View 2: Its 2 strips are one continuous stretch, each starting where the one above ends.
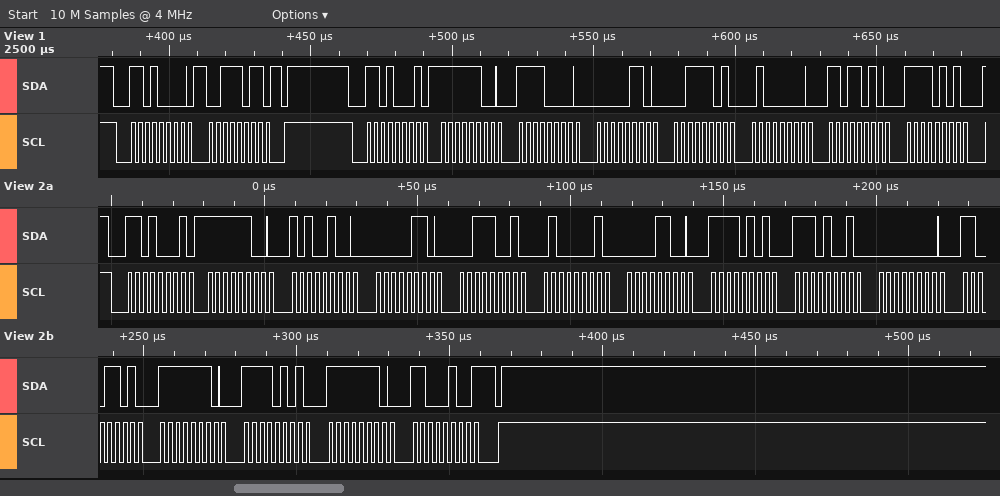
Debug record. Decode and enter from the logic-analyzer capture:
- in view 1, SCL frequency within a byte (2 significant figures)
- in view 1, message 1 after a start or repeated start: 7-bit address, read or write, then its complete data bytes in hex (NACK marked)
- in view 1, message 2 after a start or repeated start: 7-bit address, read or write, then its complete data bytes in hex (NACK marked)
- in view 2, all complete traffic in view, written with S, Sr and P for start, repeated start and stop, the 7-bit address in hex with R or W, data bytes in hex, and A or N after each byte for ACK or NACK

400 kHz
0x68 write: 3B
0x68 read: FC F0 06 3D 40 DA F5
S 68R A FC A A4 A 06 A 39 A 41 A 0C A F5 A E9 A 00 A CD A FE A F5 A FE A C4 N P
